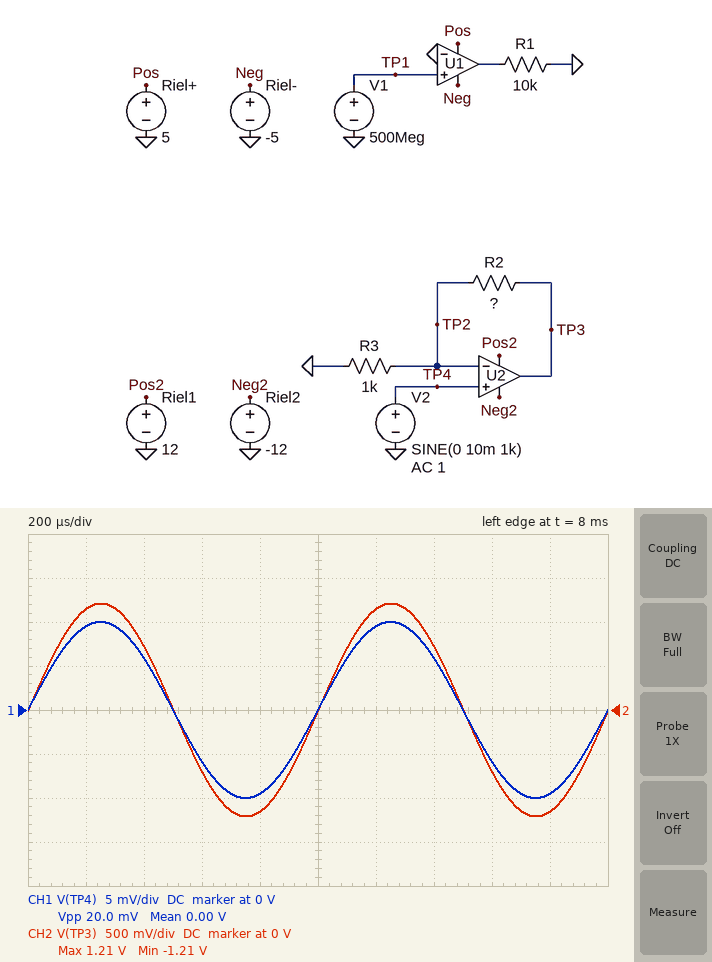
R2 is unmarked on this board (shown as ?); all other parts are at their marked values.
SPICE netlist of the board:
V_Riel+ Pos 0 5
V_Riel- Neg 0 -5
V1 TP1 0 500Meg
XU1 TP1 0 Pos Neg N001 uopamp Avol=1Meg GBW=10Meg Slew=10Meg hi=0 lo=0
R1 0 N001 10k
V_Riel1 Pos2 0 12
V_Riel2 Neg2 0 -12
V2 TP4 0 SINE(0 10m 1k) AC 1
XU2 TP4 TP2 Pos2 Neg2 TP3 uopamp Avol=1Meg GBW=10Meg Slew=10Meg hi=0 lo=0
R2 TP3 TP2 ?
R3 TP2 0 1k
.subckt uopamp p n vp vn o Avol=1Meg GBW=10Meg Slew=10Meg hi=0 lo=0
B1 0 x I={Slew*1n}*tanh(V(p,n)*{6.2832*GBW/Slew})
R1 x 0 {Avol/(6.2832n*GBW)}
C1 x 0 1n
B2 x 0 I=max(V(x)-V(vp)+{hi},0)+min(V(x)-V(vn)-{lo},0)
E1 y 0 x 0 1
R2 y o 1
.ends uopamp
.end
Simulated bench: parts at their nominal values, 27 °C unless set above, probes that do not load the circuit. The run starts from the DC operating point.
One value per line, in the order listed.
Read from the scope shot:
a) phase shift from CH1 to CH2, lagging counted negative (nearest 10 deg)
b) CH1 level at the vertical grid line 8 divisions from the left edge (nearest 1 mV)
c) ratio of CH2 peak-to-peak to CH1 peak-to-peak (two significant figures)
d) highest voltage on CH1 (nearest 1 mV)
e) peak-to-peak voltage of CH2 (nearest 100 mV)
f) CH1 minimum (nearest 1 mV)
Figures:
0 deg
-6 mV
120
10 mV
2.4 V
-10 mV
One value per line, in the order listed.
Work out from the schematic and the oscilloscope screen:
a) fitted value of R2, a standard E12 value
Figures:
120 kΩ
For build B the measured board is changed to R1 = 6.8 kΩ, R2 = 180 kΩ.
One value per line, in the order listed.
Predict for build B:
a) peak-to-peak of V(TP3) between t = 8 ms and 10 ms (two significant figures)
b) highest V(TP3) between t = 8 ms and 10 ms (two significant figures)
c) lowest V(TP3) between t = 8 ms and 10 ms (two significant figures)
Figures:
3.6 V
1.8 V
-1.8 V
